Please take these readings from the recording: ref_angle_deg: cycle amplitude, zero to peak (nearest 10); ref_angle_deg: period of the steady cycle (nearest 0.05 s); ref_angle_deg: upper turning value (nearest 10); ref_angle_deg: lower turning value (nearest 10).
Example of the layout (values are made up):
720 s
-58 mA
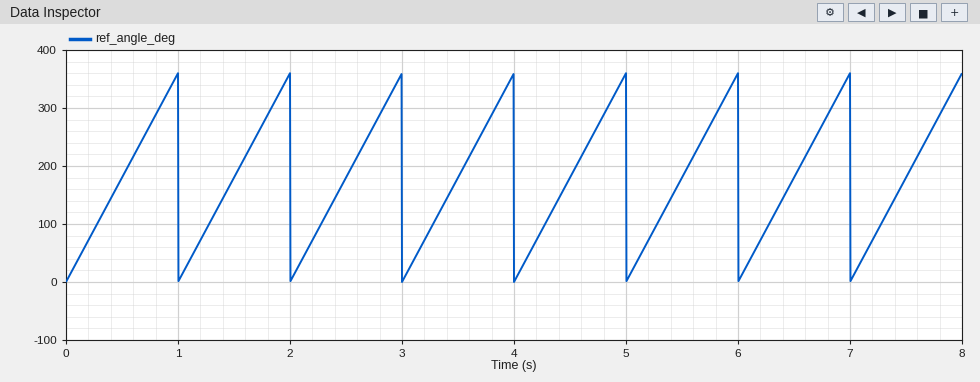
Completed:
180
1.00 s
360
0
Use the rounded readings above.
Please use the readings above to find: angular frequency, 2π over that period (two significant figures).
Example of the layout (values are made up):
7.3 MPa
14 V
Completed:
6.3 rad/s
